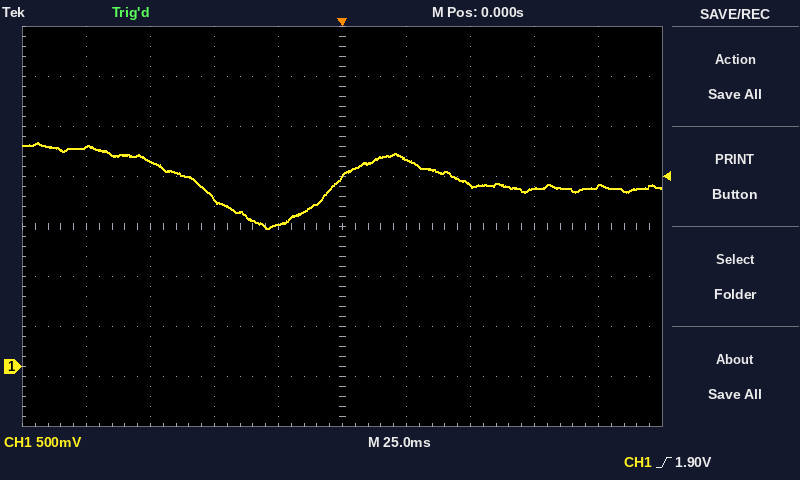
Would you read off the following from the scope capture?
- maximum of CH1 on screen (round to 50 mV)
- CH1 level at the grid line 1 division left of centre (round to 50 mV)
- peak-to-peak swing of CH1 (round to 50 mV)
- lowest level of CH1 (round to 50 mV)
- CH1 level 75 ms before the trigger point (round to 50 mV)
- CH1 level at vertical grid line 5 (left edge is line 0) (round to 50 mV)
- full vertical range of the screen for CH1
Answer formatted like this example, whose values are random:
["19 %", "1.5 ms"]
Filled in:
["2.25 V", "1.40 V", "850 mV", "1.40 V", "2.05 V", "1.90 V", "4 V"]
